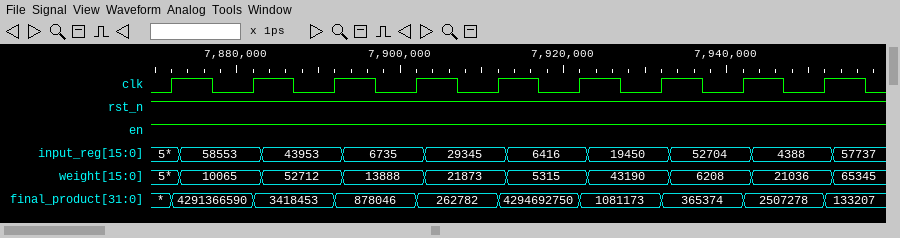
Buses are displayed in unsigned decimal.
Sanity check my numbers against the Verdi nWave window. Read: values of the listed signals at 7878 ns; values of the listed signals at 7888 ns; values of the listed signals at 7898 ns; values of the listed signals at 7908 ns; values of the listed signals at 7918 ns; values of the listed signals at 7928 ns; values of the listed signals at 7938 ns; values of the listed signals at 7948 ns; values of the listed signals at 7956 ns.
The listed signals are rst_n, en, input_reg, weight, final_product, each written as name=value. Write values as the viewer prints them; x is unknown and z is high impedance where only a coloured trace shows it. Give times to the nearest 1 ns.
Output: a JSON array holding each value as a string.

["rst_n=1, en=1, input_reg=58553, weight=10065, final_product=4291366590", "rst_n=1, en=1, input_reg=43953, weight=52712, final_product=3418453", "rst_n=1, en=1, input_reg=6735, weight=13888, final_product=878046", "rst_n=1, en=1, input_reg=29345, weight=21873, final_product=262782", "rst_n=1, en=1, input_reg=6416, weight=5315, final_product=4294692750", "rst_n=1, en=1, input_reg=19450, weight=43190, final_product=1081173", "rst_n=1, en=1, input_reg=52704, weight=6208, final_product=365374", "rst_n=1, en=1, input_reg=4388, weight=21036, final_product=2507278", "rst_n=1, en=1, input_reg=57737, weight=65345, final_product=133207"]
